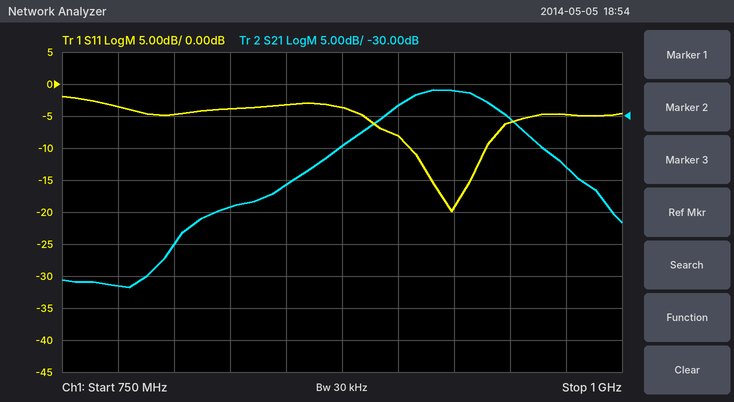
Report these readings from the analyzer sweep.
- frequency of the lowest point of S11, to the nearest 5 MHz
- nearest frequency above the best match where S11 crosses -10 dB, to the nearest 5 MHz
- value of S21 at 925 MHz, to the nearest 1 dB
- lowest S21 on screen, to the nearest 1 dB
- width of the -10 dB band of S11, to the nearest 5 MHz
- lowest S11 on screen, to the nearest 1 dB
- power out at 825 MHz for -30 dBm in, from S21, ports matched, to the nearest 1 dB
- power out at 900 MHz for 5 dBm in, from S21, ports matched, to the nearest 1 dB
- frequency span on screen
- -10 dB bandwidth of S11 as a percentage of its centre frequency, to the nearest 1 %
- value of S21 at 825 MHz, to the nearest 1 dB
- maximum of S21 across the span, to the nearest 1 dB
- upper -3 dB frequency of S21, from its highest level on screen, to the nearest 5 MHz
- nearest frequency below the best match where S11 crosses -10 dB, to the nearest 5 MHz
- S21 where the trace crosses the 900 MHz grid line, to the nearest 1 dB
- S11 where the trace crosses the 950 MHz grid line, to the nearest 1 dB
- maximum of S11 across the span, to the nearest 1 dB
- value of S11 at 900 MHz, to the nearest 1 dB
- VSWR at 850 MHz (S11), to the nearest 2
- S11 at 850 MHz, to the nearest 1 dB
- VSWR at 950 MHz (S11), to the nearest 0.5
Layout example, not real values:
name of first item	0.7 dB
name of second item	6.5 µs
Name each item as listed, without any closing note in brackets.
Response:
frequency of the lowest point of S11, to the nearest 5 MHz	925 MHz
nearest frequency above the best match where S11 crosses -10 dB, to the nearest 5 MHz	940 MHz
value of S21 at 925 MHz, to the nearest 1 dB	-26 dB
lowest S21 on screen, to the nearest 1 dB	-57 dB
width of the -10 dB band of S11, to the nearest 5 MHz	35 MHz
lowest S11 on screen, to the nearest 1 dB	-20 dB
power out at 825 MHz for -30 dBm in, from S21, ports matched, to the nearest 1 dB	-74 dBm
power out at 900 MHz for 5 dBm in, from S21, ports matched, to the nearest 1 dB	-23 dBm
frequency span on screen	250 MHz
-10 dB bandwidth of S11 as a percentage of its centre frequency, to the nearest 1 %	4 %
value of S21 at 825 MHz, to the nearest 1 dB	-44 dB
maximum of S21 across the span, to the nearest 1 dB	-26 dB
upper -3 dB frequency of S21, from its highest level on screen, to the nearest 5 MHz	945 MHz
nearest frequency below the best match where S11 crosses -10 dB, to the nearest 5 MHz	905 MHz
S21 where the trace crosses the 900 MHz grid line, to the nearest 1 dB	-28 dB
S11 where the trace crosses the 950 MHz grid line, to the nearest 1 dB	-6 dB
maximum of S11 across the span, to the nearest 1 dB	-2 dB
value of S11 at 900 MHz, to the nearest 1 dB	-8 dB
VSWR at 850 MHz (S11), to the nearest 2	6
S11 at 850 MHz, to the nearest 1 dB	-3 dB
VSWR at 950 MHz (S11), to the nearest 0.5	3.0
